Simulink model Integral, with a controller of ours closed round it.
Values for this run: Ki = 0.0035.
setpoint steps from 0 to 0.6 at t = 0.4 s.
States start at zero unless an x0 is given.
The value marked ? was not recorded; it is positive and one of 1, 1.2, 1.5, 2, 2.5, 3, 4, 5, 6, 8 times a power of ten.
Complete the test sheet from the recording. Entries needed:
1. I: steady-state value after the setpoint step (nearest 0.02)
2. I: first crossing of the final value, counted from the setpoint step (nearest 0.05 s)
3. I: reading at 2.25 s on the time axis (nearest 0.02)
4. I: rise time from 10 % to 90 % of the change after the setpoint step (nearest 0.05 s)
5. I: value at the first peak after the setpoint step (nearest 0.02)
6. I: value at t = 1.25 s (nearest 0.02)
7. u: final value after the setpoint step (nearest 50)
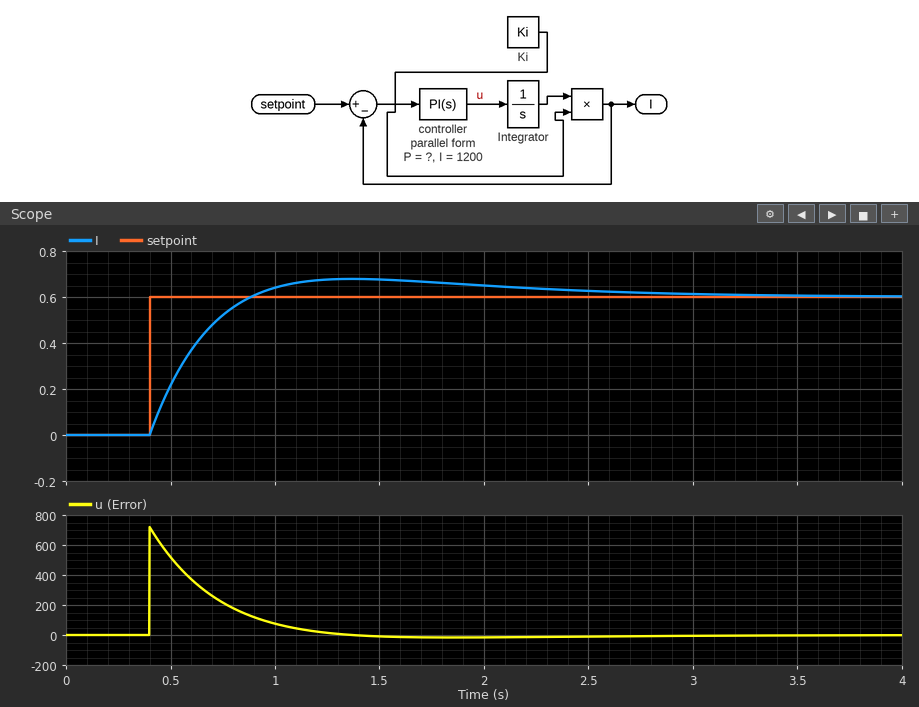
0.60
0.50 s
0.64
0.35 s
0.68
0.68
0
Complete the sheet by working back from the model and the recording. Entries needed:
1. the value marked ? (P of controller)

1200
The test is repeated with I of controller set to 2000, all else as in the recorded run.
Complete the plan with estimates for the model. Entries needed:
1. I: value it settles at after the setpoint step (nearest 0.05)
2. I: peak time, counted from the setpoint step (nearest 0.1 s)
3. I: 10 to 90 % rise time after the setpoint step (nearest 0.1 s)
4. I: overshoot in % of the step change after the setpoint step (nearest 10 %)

0.60
0.8 s
0.3 s
20 %
